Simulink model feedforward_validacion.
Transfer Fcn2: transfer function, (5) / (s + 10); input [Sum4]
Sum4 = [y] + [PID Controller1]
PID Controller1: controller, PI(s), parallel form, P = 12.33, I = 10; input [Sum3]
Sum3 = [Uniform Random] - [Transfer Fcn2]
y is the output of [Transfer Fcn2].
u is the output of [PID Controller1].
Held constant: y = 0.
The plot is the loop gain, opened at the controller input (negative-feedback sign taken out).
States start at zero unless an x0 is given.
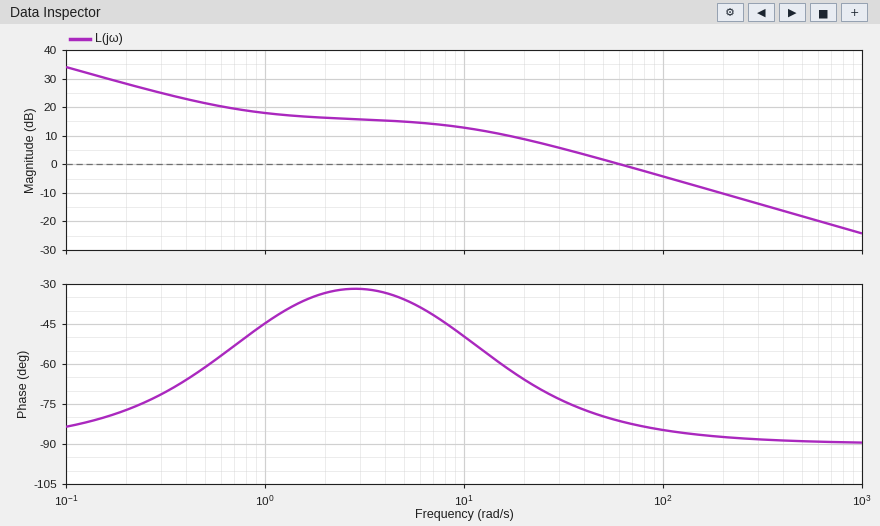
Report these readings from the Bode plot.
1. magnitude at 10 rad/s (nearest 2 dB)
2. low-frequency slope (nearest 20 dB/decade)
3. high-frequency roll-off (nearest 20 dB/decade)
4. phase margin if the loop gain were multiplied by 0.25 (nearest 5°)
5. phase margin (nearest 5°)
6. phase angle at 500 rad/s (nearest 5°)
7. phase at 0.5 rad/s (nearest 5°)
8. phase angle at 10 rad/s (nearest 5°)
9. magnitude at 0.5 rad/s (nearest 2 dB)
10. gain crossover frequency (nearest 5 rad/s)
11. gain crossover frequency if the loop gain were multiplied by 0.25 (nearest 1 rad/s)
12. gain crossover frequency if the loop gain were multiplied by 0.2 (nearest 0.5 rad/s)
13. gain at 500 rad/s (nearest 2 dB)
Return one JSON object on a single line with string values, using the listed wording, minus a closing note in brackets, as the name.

{"magnitude at 10 rad/s": "12 dB", "low-frequency slope": "-20 dB/decade", "high-frequency roll-off": "-20 dB/decade", "phase margin if the loop gain were multiplied by 0.25": "125°", "phase margin": "100°", "phase angle at 500 rad/s": "-90°", "phase at 0.5 rad/s": "-60°", "phase angle at 10 rad/s": "-50°", "magnitude at 0.5 rad/s": "22 dB", "gain crossover frequency": "60 rad/s", "gain crossover frequency if the loop gain were multiplied by 0.25": "12 rad/s", "gain crossover frequency if the loop gain were multiplied by 0.2": "7.5 rad/s", "gain at 500 rad/s": "-18 dB"}
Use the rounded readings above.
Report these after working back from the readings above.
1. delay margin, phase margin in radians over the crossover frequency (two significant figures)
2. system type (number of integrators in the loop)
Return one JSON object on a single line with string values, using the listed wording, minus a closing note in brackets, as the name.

{"delay margin, phase margin in radians over the crossover frequency": "0.029 s", "system type": "1"}
